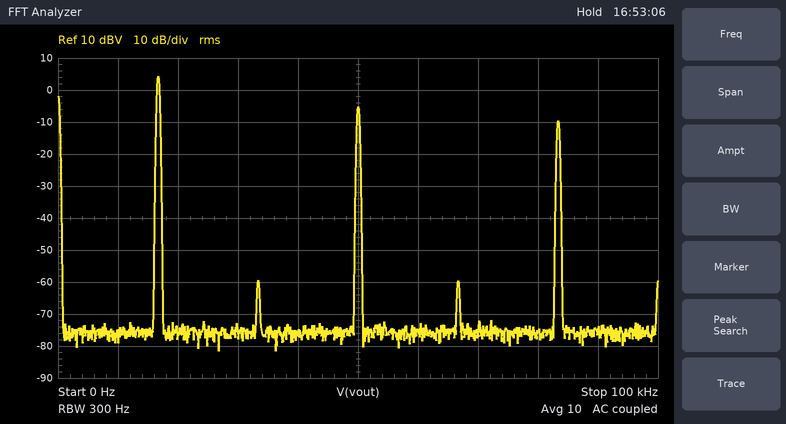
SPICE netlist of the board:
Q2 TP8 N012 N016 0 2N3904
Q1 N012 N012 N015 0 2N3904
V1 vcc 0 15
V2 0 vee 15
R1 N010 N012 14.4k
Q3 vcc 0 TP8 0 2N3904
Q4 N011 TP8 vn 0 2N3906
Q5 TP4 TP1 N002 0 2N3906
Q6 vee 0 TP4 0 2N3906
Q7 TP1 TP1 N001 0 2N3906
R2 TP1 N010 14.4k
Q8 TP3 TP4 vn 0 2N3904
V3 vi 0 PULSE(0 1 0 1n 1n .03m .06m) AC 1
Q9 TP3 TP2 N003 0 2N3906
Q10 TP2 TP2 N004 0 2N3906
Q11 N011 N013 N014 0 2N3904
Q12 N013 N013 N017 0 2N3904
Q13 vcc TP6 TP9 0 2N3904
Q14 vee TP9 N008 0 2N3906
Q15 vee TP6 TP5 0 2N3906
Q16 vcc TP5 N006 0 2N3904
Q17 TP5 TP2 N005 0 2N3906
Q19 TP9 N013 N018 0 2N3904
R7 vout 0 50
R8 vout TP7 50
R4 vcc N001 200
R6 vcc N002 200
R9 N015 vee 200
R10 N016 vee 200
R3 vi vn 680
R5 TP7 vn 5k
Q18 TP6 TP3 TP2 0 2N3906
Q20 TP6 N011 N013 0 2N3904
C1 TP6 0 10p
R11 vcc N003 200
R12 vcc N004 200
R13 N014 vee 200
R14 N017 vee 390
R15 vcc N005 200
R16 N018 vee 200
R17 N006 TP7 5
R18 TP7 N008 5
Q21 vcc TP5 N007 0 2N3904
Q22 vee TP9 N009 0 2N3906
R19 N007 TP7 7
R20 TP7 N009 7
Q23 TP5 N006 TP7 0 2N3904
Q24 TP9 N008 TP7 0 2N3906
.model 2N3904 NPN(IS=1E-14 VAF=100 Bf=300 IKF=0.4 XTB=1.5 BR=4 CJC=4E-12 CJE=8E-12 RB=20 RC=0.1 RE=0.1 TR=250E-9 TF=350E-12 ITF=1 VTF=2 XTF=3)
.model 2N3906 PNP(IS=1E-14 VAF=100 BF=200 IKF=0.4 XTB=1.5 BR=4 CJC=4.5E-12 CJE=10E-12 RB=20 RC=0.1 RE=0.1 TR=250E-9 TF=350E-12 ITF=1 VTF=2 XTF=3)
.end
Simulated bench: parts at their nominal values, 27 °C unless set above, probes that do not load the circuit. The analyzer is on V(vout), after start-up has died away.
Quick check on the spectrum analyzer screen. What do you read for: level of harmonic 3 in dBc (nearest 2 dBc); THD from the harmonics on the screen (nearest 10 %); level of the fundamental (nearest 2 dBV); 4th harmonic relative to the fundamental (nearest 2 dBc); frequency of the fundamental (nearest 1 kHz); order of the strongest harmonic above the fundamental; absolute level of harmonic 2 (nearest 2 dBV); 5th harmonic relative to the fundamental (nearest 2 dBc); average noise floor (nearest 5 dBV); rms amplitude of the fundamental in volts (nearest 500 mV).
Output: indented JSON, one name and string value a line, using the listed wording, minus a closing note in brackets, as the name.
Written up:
{
  "level of harmonic 3 in dBc": "-10 dBc",
  "THD from the harmonics on the screen": "40 %",
  "level of the fundamental": "4 dBV",
  "4th harmonic relative to the fundamental": "-64 dBc",
  "frequency of the fundamental": "17 kHz",
  "order of the strongest harmonic above the fundamental": "3",
  "absolute level of harmonic 2": "-60 dBV",
  "5th harmonic relative to the fundamental": "-14 dBc",
  "average noise floor": "-75 dBV",
  "rms amplitude of the fundamental in volts": "1.5 V"
}
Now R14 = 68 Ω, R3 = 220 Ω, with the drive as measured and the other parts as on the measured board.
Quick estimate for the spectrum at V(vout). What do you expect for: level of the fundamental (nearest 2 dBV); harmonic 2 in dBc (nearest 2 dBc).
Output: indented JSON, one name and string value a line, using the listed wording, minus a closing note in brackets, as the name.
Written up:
{
  "level of the fundamental": "6 dBV",
  "harmonic 2 in dBc": "-22 dBc"
}
